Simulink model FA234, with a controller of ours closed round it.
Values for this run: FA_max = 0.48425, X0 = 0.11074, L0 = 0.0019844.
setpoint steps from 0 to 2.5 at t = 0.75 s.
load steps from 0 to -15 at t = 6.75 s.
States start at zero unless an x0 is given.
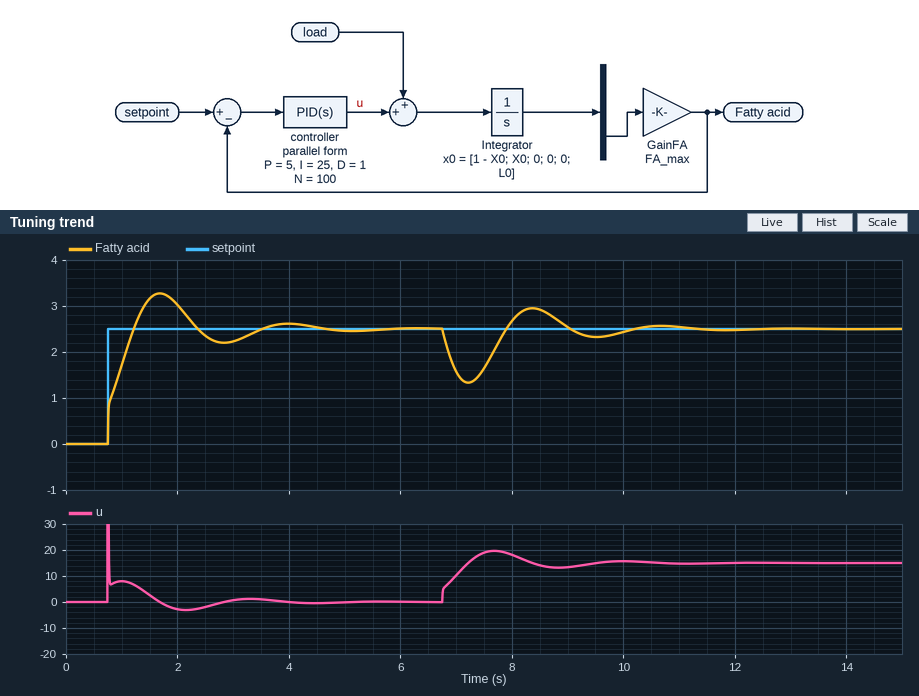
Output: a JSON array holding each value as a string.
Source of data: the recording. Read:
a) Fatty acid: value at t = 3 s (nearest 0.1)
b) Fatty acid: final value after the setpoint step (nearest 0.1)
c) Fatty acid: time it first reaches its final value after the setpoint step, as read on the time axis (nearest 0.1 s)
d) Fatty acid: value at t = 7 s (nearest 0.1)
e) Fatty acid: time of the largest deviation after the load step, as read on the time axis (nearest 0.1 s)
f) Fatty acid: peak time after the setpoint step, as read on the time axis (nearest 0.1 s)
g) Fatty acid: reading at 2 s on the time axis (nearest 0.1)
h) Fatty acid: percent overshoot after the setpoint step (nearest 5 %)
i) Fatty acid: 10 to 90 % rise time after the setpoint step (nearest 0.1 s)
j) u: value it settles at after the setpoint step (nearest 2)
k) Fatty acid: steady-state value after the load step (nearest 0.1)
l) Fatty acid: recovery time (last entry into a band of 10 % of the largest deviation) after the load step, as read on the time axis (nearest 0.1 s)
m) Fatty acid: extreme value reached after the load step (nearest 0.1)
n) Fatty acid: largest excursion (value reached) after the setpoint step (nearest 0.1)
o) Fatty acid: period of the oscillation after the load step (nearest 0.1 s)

["2.2", "2.5", "1.2 s", "1.6", "7.2 s", "1.7 s", "3.0", "30 %", "0.4 s", "0", "2.5", "9.8 s", "1.3", "3.3", "2.3 s"]
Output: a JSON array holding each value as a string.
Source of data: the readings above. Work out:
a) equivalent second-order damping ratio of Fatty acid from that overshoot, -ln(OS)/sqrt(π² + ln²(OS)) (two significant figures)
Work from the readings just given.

["0.36"]
